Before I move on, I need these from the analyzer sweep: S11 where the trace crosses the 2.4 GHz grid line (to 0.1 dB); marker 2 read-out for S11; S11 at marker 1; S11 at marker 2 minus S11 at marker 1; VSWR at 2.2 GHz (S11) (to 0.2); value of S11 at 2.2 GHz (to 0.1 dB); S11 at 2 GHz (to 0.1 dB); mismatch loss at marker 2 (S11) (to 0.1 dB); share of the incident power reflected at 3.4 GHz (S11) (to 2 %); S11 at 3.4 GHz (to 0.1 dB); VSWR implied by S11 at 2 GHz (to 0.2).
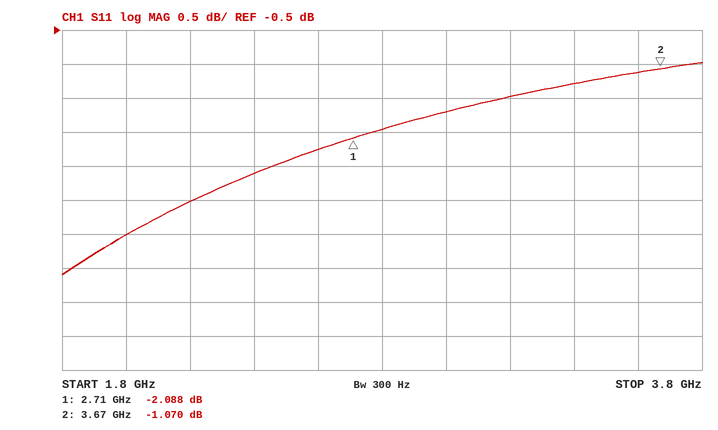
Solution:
-2.6 dB
-1.070 dB
-2.088 dB
1.018 dB
5.8
-3.0 dB
-3.5 dB
6.6 dB
74 %
-1.3 dB
5.0
